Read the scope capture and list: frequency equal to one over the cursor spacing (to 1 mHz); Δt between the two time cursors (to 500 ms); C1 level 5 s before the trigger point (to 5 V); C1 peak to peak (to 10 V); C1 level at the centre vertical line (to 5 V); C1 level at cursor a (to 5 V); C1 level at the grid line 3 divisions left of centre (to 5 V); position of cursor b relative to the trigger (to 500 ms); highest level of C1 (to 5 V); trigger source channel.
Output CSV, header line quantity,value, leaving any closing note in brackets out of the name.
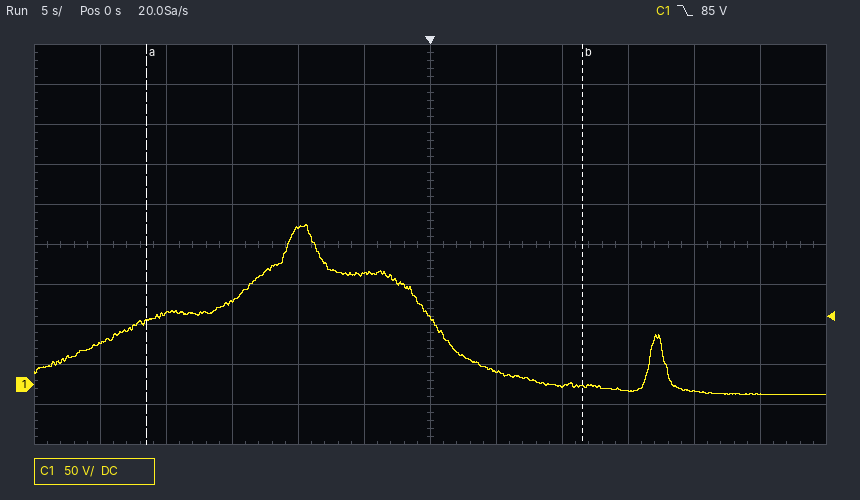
quantity,value
frequency equal to one over the cursor spacing,30 mHz
Δt between the two time cursors,33.0 s
C1 level 5 s before the trigger point,140 V
C1 peak to peak,210 V
C1 level at the centre vertical line,85 V
C1 level at cursor a,80 V
C1 level at the grid line 3 divisions left of centre,105 V
position of cursor b relative to the trigger,+11.5 s
highest level of C1,200 V
trigger source channel,C1
